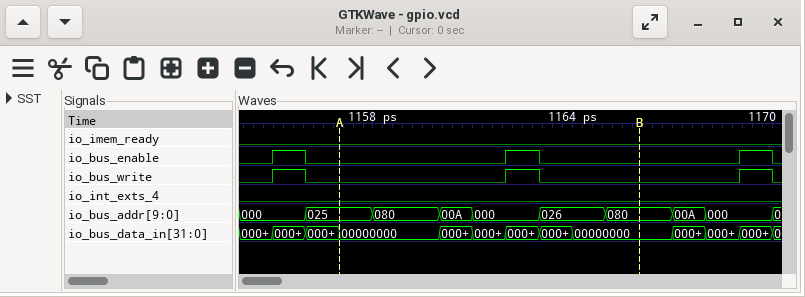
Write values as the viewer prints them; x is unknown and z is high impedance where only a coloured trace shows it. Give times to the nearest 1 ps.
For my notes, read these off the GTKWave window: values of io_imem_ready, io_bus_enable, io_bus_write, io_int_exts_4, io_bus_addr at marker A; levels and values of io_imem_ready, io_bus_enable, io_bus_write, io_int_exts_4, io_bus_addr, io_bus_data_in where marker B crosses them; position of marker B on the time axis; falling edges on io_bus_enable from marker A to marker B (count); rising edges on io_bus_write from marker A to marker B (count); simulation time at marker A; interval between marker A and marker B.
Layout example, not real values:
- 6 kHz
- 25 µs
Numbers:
- io_imem_ready=0, io_bus_enable=0, io_bus_write=0, io_int_exts_4=0, io_bus_addr=025
- io_imem_ready=0, io_bus_enable=0, io_bus_write=0, io_int_exts_4=0, io_bus_addr=080, io_bus_data_in=00000000
- 1166 ps
- 1
- 1
- 1157 ps
- 9 ps
